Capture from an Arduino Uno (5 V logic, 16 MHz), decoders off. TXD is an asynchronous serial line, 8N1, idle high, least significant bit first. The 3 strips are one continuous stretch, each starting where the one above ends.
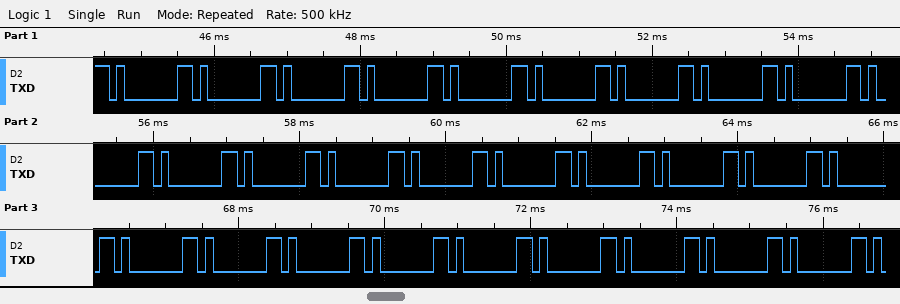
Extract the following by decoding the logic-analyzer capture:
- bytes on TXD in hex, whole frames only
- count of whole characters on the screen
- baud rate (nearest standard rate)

01 01 01 01 01 01 01 01 01 01 01 01 01 01 01 01 01 01 01 01 01 01 01 01 01 01 01 01
28
9600 baud
